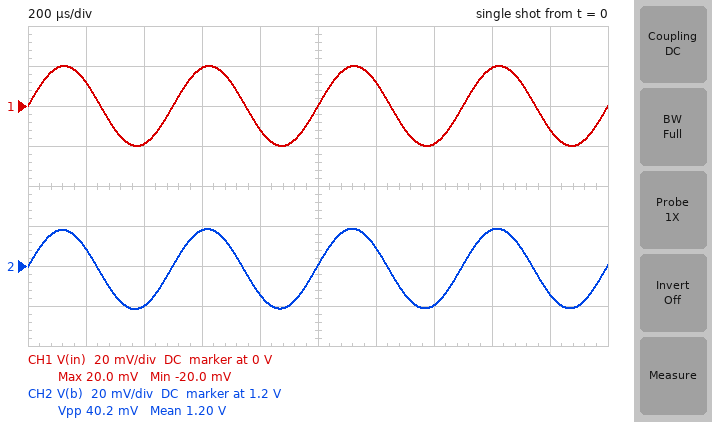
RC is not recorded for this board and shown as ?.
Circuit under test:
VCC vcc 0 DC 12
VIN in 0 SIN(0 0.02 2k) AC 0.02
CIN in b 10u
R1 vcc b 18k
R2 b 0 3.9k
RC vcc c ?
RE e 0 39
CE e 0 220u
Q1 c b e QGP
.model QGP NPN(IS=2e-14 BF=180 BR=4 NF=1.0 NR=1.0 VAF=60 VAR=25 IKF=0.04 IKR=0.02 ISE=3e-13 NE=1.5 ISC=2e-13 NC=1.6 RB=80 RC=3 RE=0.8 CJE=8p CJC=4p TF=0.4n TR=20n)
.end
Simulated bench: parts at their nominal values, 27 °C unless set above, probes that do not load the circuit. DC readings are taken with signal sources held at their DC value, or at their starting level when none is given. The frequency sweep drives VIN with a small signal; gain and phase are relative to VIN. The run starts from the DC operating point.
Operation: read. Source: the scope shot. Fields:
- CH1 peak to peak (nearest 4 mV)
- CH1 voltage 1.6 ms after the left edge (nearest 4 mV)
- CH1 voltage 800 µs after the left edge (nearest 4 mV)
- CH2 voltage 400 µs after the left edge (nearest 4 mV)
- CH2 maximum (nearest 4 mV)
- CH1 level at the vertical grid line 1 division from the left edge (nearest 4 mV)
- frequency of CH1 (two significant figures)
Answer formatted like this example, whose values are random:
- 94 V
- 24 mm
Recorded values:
- 40 mV
- 20 mV
- -12 mV
- 1.180 V
- 1.220 V
- 12 mV
- 2.0 kHz
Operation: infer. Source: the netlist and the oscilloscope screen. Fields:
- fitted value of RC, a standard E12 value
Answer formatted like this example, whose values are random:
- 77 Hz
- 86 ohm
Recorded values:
- 1 kΩ
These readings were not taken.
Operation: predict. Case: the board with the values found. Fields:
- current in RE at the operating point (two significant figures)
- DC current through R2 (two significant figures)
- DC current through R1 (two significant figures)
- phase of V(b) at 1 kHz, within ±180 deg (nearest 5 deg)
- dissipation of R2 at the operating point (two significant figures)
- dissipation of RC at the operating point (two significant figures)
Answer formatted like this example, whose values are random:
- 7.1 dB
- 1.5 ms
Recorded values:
- 12 mA
- 310 µA
- 600 µA
- 10 deg
- 370 µW
- 130 mW
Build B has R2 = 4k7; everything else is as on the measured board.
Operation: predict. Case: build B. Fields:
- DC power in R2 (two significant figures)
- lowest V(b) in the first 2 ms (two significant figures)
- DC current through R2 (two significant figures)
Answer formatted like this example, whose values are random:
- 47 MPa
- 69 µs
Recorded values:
- 310 µW
- 1.2 V
- 260 µA
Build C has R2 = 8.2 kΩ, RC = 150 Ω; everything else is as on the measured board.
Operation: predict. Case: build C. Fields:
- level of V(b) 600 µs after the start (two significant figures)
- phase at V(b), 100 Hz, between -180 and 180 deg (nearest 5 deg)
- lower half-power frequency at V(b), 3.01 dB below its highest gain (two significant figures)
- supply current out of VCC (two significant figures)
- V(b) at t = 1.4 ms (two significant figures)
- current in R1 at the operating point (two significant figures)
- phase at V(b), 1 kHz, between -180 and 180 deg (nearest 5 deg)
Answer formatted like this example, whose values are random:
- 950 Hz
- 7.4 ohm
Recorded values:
- 2.0 V
- 10 deg
- 15 Hz
- 30 mA
- 1.9 V
- 560 µA
- 5 deg
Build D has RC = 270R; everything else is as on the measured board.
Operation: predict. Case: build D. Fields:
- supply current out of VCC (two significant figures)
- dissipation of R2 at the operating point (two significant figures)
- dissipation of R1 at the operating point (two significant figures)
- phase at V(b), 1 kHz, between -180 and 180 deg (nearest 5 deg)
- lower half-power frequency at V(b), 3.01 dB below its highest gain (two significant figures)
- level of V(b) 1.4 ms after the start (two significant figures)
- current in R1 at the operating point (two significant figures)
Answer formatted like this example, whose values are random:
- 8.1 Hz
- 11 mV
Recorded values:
- 20 mA
- 600 µW
- 6.1 mW
- 5 deg
- 14 Hz
- 1.5 V
- 580 µA
